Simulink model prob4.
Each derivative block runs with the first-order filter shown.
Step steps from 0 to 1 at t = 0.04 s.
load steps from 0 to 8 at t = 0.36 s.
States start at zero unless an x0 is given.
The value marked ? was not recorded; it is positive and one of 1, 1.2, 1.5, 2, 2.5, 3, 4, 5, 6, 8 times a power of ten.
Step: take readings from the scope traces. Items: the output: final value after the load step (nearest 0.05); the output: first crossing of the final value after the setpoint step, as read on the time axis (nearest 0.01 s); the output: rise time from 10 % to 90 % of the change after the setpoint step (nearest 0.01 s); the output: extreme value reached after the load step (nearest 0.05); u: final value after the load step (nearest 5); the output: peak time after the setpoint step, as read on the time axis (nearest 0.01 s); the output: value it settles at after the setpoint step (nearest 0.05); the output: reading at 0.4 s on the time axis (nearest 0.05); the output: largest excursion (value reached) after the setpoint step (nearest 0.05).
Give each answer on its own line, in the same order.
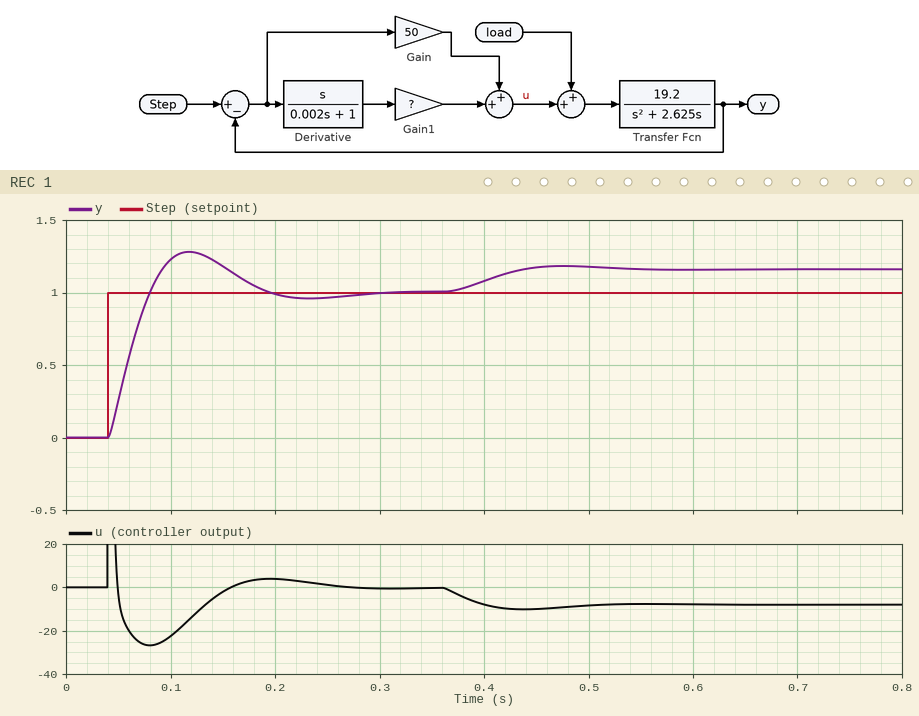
1.15
0.08 s
0.03 s
1.20
-10
0.12 s
1.00
1.10
1.30
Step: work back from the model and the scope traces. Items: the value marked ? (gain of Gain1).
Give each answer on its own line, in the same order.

1.5
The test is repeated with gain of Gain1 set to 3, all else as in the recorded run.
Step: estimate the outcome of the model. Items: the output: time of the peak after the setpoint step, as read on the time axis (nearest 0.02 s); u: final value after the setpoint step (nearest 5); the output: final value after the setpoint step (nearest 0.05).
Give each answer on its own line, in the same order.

0.10 s
0
1.00
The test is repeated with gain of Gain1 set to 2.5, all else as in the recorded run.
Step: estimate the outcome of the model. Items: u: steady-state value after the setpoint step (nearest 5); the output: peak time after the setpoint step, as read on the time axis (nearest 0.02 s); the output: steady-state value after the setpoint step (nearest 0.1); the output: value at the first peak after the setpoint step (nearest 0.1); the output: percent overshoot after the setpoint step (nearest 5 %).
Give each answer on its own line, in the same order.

0
0.10 s
1.0
1.2
15 %
